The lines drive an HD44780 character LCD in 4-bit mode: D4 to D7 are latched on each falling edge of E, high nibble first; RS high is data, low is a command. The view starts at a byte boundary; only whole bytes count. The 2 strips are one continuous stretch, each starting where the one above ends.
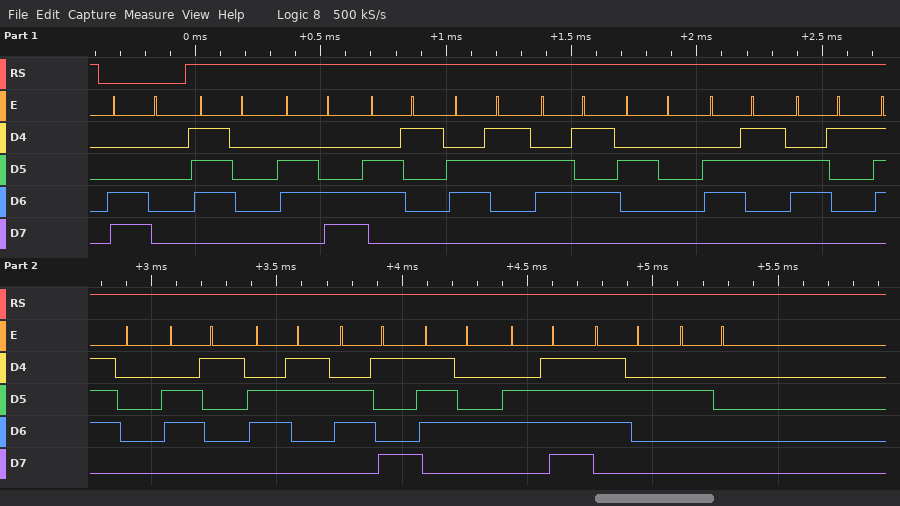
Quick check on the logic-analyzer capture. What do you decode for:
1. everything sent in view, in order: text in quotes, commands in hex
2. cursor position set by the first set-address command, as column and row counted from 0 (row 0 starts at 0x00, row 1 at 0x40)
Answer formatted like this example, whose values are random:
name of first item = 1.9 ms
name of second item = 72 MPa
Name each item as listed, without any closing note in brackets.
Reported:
everything sent in view, in order: text in quotes, commands in hex = 0xC0 "place capacitor "
cursor position set by the first set-address command, as column and row counted from 0 = column 0, row 1
